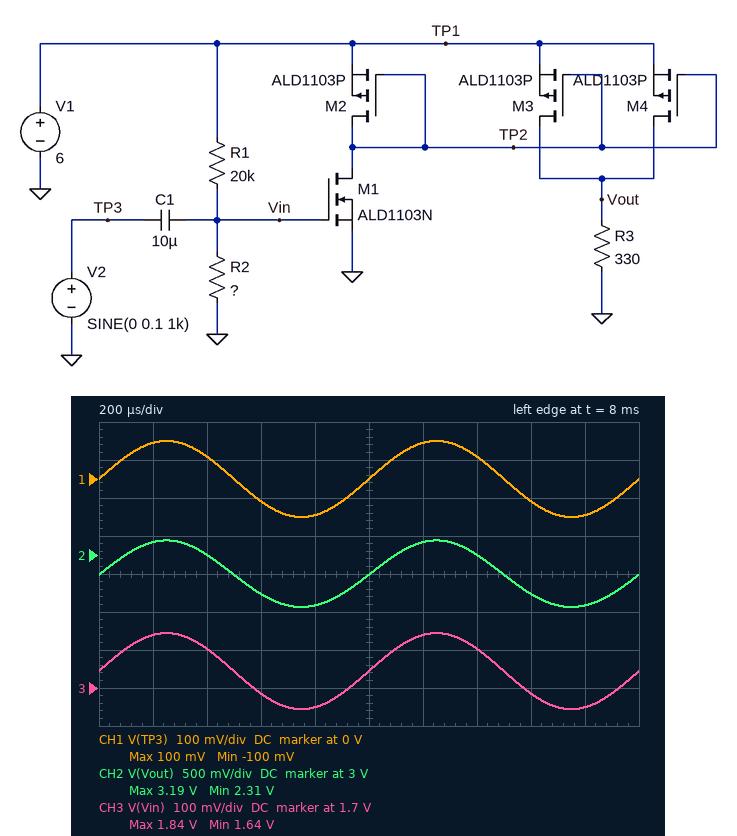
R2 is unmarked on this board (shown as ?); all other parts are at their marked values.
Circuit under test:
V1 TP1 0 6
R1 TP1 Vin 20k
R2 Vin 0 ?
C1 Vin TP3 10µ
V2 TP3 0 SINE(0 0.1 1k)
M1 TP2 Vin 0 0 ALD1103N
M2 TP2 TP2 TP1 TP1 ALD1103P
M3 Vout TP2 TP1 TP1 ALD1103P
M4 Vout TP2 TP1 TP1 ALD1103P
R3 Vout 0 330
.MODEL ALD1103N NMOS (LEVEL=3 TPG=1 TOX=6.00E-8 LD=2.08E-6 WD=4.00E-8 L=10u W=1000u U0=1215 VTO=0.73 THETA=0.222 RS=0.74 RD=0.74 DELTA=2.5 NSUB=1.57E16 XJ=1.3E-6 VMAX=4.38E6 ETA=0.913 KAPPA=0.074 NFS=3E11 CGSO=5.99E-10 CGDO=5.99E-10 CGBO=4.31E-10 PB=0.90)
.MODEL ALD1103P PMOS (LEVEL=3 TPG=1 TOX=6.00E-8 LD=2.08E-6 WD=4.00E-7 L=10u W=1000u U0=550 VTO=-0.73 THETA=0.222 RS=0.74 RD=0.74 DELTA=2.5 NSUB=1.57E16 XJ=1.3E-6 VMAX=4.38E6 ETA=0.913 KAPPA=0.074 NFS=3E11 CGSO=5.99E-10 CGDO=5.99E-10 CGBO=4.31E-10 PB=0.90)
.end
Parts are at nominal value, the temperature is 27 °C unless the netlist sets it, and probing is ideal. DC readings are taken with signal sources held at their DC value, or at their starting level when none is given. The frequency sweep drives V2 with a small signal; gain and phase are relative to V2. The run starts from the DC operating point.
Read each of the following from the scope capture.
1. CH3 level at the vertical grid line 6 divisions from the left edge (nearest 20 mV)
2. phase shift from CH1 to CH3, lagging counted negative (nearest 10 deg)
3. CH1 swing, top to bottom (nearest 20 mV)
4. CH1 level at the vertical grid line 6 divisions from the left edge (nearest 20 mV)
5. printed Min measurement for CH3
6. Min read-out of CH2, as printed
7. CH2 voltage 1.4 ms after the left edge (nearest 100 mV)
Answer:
1.84 V
0 deg
200 mV
100 mV
1.64 V
2.31 V
3.0 V
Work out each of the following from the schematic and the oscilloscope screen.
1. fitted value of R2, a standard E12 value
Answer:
8.2 kΩ
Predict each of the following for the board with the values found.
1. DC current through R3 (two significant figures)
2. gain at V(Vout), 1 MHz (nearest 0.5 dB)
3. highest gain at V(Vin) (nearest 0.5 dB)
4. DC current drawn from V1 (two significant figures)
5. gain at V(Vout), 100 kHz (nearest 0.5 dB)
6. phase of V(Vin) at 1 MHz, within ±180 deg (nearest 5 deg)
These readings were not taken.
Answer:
8.3 mA
13.0 dB
0 dB
13 mA
13.0 dB
0 deg
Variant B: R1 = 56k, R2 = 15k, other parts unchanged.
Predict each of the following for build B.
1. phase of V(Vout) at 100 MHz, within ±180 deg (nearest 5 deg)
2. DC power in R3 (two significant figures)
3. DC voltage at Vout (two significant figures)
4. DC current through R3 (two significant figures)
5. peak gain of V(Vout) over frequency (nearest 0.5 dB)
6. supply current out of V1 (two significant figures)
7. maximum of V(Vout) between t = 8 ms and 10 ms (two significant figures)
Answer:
-95 deg
3.0 mW
990 mV
3.0 mA
9.0 dB
4.5 mA
1.3 V
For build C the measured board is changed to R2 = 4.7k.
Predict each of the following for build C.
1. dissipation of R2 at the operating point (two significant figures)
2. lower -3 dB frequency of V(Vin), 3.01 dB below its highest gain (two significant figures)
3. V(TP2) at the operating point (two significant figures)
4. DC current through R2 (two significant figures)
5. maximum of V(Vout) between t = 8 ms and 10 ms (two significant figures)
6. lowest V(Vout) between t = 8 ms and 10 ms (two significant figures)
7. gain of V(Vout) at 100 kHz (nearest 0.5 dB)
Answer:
280 µW
4.2 Hz
4.6 V
240 µA
920 mV
440 mV
7.5 dB
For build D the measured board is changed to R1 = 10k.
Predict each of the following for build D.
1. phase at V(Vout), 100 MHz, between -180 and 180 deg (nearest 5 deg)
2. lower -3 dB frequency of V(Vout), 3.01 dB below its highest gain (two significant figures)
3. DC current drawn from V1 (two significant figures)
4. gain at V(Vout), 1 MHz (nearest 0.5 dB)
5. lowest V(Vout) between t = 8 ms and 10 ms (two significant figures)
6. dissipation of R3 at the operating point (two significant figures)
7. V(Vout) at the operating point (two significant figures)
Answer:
-95 deg
3.5 Hz
28 mA
-7.5 dB
5.0 V
78 mW
5.1 V
